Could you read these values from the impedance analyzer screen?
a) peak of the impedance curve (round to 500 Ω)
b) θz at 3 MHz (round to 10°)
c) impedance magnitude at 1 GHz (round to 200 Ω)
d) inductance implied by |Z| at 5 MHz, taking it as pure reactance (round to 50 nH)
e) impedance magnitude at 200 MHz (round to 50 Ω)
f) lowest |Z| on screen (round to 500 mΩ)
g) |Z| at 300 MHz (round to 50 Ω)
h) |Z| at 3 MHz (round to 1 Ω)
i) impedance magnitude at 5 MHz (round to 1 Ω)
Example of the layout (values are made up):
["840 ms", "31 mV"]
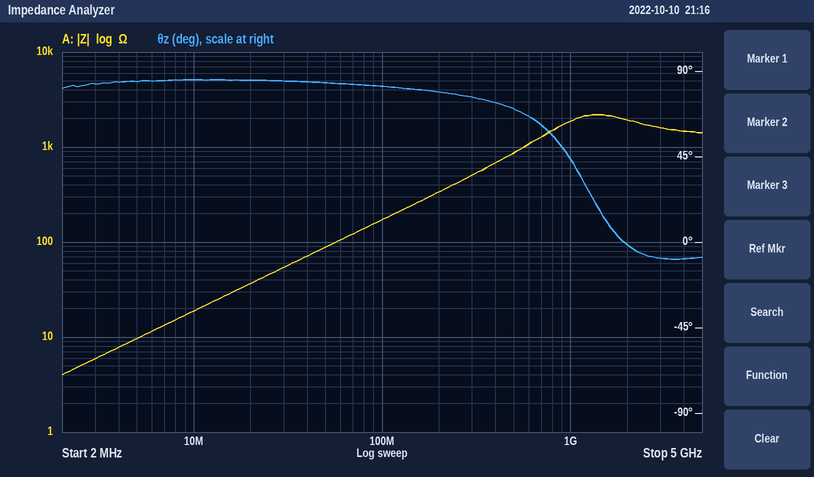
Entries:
["2.0 kΩ", "80°", "1.8 kΩ", "300 nH", "350 Ω", "4.0 Ω", "500 Ω", "6 Ω", "10 Ω"]
